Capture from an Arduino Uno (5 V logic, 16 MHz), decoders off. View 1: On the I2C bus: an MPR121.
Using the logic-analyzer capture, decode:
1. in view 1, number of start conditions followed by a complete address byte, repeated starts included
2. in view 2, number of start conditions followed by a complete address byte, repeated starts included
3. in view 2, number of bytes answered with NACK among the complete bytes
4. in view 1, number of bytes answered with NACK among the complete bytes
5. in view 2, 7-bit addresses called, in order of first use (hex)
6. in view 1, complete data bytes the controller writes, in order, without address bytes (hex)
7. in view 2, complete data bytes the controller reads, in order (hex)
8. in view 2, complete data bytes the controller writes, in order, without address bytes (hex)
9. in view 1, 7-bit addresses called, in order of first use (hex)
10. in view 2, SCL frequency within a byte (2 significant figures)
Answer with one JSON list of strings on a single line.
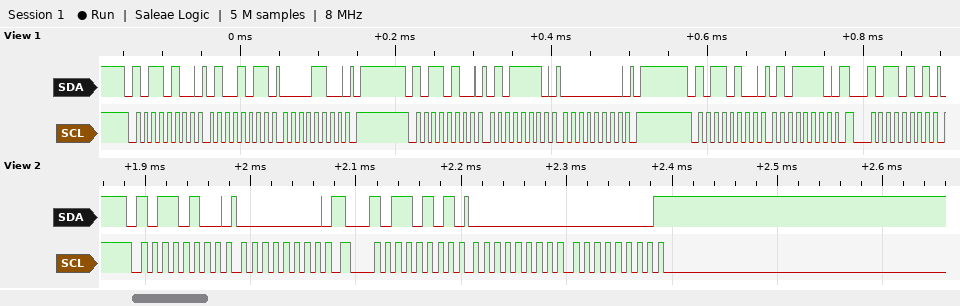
["4", "2", "1", "0", "0x5A", "4B 0C 5E 00 5E", "00 00", "00", "0x5A", "100 kHz"]
